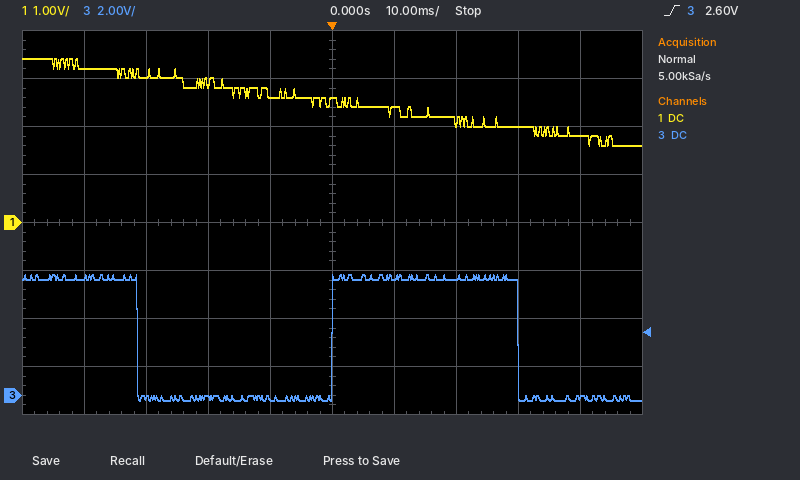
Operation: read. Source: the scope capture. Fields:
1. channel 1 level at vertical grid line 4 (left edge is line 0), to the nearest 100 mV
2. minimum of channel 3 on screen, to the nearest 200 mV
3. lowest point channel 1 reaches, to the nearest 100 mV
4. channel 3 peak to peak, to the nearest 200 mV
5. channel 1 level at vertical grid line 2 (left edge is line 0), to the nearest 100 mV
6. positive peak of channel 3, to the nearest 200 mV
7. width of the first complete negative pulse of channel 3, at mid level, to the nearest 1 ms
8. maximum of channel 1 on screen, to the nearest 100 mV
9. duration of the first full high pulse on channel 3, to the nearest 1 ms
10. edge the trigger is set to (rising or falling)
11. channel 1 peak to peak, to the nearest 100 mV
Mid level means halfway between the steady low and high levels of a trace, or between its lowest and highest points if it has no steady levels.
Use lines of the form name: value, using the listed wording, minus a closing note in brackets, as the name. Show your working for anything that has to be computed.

channel 1 level at vertical grid line 4 (left edge is line 0), to the nearest 100 mV: 2.7 V
minimum of channel 3 on screen, to the nearest 200 mV: -200 mV
lowest point channel 1 reaches, to the nearest 100 mV: 1.6 V
channel 3 peak to peak, to the nearest 200 mV: 5.0 V − (-200 mV) = 5.2 V
channel 1 level at vertical grid line 2 (left edge is line 0), to the nearest 100 mV: 3.1 V
positive peak of channel 3, to the nearest 200 mV: 5.0 V
width of the first complete negative pulse of channel 3, at mid level, to the nearest 1 ms: 31 ms
maximum of channel 1 on screen, to the nearest 100 mV: 3.4 V
duration of the first full high pulse on channel 3, to the nearest 1 ms: 30 ms
edge the trigger is set to: rising
channel 1 peak to peak, to the nearest 100 mV: 3.4 V − (1.6 V) = 1.8 V
